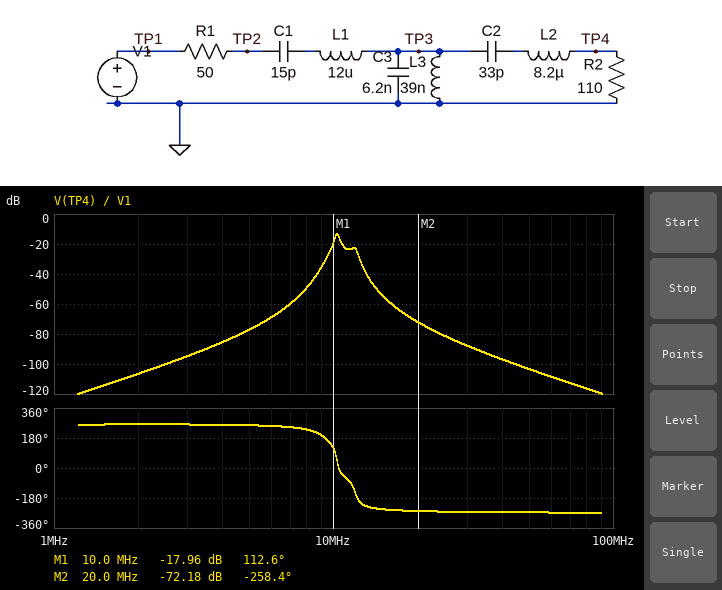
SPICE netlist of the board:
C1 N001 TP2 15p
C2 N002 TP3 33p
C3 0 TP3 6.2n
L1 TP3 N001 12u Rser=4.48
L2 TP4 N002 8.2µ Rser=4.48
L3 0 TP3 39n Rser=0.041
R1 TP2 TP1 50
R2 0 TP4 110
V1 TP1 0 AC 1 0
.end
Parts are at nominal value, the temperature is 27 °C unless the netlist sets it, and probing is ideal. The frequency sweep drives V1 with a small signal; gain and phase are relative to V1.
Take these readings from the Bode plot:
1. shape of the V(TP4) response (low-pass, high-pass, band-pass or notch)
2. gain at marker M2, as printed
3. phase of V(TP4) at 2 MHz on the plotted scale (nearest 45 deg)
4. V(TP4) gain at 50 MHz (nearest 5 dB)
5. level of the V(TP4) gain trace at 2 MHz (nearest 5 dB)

band-pass
-72.18 dB
270 deg
-105 dB
-105 dB
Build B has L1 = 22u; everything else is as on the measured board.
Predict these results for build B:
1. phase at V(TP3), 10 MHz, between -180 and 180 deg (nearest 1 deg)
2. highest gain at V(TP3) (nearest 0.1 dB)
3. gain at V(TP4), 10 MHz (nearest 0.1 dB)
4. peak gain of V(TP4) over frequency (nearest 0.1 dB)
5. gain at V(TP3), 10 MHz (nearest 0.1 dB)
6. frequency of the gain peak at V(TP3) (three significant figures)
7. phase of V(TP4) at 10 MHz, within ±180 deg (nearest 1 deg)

-23 deg
-14.6 dB
-20.0 dB
-16.1 dB
-19.3 dB
10.3 MHz
-39 deg
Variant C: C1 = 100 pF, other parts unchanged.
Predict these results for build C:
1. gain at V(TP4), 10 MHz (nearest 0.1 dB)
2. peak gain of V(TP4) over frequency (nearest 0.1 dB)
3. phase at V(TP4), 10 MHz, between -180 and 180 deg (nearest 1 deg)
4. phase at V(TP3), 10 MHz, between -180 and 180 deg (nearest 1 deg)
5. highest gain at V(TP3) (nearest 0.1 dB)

-24.8 dB
-19.9 dB
-45 deg
-29 deg
-18.4 dB
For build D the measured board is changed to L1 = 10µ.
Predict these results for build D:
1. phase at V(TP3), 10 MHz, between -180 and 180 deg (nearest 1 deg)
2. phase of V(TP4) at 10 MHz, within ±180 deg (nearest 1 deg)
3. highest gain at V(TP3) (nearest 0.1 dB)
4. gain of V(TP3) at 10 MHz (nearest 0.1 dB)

133 deg
117 deg
-14.7 dB
-20.4 dB
